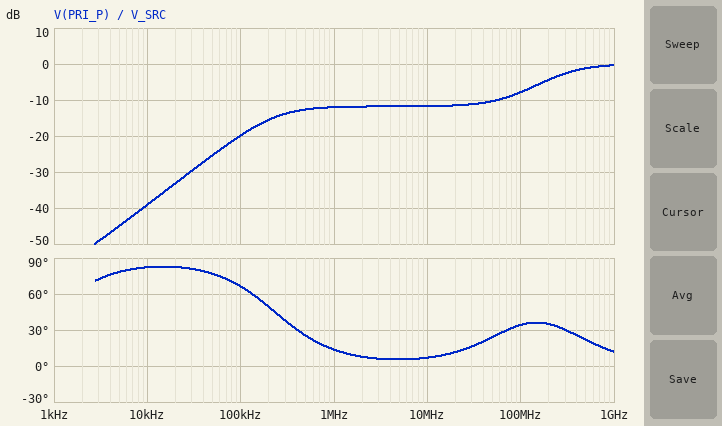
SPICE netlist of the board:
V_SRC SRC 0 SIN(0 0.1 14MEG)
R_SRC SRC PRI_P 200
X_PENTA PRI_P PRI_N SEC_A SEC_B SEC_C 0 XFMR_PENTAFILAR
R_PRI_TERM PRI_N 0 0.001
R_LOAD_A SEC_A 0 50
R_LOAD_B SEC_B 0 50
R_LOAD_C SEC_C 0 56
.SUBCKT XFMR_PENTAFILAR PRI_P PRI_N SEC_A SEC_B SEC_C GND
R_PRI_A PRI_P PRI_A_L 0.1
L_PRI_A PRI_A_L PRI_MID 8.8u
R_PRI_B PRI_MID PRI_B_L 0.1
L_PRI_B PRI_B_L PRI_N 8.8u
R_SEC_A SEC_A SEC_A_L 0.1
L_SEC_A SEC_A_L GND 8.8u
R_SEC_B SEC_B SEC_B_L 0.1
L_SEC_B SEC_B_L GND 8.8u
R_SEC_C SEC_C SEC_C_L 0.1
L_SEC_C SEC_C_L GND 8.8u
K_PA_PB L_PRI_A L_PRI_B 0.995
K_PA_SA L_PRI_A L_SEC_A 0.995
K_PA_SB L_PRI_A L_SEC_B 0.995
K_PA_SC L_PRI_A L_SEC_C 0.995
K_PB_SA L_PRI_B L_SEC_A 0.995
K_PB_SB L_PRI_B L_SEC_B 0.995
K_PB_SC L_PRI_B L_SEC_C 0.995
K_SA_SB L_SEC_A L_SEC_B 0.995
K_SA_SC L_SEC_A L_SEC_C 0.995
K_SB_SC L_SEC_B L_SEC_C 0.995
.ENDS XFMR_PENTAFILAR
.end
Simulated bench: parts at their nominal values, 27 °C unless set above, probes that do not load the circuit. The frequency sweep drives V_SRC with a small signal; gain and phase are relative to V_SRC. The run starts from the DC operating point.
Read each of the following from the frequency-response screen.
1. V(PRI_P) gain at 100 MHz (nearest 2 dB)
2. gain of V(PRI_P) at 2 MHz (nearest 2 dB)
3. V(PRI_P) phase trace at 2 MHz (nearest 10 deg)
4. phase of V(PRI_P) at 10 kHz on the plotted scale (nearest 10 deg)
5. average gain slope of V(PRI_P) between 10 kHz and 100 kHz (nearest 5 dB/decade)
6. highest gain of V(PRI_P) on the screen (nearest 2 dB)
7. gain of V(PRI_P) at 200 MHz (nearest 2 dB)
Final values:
-8 dB
-12 dB
10 deg
80 deg
20 dB/decade
0 dB
-4 dB
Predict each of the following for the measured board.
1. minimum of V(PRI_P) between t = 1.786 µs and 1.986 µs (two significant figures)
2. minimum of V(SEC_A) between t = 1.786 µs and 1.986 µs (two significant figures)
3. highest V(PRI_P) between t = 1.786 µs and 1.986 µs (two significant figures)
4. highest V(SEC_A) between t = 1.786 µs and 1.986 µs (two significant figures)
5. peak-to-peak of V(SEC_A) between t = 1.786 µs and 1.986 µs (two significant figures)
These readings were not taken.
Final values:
-26 mV
-13 mV
26 mV
13 mV
26 mV
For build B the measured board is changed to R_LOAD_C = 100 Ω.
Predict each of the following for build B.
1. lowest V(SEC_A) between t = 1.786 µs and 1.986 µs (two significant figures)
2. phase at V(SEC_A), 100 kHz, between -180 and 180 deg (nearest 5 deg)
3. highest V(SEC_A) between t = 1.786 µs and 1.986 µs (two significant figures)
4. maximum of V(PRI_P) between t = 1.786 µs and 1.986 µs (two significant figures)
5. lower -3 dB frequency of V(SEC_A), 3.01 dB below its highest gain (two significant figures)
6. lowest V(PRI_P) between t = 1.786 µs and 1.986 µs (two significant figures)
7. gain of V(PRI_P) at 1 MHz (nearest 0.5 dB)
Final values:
-14 mV
70 deg
14 mV
29 mV
260 kHz
-29 mV
-11.0 dB
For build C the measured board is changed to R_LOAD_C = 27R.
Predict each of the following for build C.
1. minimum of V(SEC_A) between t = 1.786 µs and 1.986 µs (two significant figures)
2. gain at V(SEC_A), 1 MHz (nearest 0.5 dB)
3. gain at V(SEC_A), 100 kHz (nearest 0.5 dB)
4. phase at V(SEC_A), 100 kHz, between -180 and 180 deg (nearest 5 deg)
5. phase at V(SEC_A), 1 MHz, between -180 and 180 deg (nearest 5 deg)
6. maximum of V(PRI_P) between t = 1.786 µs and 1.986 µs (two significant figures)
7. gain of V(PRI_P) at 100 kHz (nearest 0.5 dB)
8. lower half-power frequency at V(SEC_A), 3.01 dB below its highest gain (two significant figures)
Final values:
-10 mV
-20.0 dB
-26.5 dB
60 deg
10 deg
21 mV
-20.0 dB
200 kHz
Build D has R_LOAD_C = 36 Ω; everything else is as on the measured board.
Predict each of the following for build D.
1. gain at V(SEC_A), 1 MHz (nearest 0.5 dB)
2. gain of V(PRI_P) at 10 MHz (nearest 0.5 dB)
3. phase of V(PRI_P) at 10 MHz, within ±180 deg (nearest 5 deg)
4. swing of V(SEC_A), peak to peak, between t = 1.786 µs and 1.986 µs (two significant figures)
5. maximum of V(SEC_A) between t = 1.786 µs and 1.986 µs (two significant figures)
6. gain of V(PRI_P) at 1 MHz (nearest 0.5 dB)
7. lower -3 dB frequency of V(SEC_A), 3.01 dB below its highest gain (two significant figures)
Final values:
-19.0 dB
-12.5 dB
10 deg
23 mV
11 mV
-13.0 dB
210 kHz
